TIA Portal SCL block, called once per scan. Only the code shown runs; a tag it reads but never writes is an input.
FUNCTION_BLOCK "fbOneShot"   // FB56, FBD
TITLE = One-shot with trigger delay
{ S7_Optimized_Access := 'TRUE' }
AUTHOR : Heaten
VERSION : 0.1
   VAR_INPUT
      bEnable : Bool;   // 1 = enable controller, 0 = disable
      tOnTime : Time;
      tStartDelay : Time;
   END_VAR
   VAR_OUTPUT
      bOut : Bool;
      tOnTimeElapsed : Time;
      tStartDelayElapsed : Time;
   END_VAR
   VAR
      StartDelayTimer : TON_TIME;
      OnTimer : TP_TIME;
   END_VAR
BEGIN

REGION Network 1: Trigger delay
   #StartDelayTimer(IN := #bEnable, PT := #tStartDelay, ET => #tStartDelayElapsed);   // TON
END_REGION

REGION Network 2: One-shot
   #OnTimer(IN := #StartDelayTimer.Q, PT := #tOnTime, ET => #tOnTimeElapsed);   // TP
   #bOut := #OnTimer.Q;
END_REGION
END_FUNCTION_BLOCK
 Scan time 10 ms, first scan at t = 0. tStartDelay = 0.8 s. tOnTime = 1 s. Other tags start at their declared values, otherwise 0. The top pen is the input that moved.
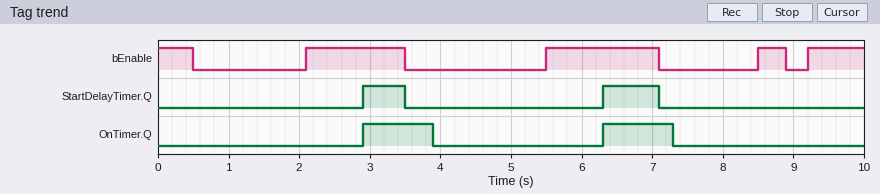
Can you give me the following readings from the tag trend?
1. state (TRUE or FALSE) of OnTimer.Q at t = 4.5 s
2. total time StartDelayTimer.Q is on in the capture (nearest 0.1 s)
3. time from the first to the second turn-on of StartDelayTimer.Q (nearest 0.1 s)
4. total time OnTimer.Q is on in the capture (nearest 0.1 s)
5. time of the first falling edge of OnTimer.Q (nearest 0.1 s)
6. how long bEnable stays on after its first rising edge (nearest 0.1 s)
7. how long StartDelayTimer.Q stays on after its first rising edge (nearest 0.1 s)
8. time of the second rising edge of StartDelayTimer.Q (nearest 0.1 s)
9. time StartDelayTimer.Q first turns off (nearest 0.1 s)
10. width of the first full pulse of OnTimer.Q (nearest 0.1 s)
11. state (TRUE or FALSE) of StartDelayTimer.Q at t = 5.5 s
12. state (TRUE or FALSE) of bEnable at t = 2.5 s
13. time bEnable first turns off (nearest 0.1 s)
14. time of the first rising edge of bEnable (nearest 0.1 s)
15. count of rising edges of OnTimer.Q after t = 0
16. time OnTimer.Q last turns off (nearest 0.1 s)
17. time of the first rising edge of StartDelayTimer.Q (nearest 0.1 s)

FALSE
1.4 s
3.4 s
2.0 s
3.9 s
1.4 s
0.6 s
6.3 s
3.5 s
1.0 s
FALSE
TRUE
0.5 s
2.1 s
2
7.3 s
2.9 s
